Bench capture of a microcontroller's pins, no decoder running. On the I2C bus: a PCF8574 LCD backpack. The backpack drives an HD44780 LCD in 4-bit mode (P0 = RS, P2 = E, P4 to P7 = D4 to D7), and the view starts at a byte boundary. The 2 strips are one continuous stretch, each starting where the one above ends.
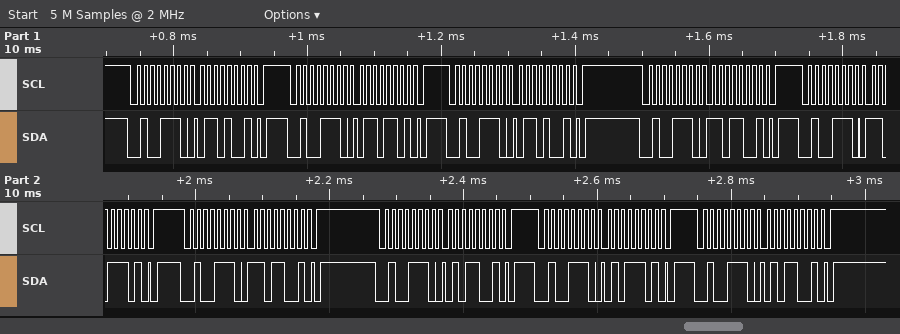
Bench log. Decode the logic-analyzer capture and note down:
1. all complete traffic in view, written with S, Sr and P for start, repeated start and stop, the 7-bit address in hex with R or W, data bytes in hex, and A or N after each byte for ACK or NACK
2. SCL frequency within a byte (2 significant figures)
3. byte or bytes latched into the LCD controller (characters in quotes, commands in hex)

S 27W A 69 A P S 27W A 6D A P S 27W A 69 A P S 27W A D9 A P S 27W A DD A P S 27W A D9 A P S 27W A 59 A P S 27W A 5D A P S 27W A 59 A P
100 kHz
'm'
